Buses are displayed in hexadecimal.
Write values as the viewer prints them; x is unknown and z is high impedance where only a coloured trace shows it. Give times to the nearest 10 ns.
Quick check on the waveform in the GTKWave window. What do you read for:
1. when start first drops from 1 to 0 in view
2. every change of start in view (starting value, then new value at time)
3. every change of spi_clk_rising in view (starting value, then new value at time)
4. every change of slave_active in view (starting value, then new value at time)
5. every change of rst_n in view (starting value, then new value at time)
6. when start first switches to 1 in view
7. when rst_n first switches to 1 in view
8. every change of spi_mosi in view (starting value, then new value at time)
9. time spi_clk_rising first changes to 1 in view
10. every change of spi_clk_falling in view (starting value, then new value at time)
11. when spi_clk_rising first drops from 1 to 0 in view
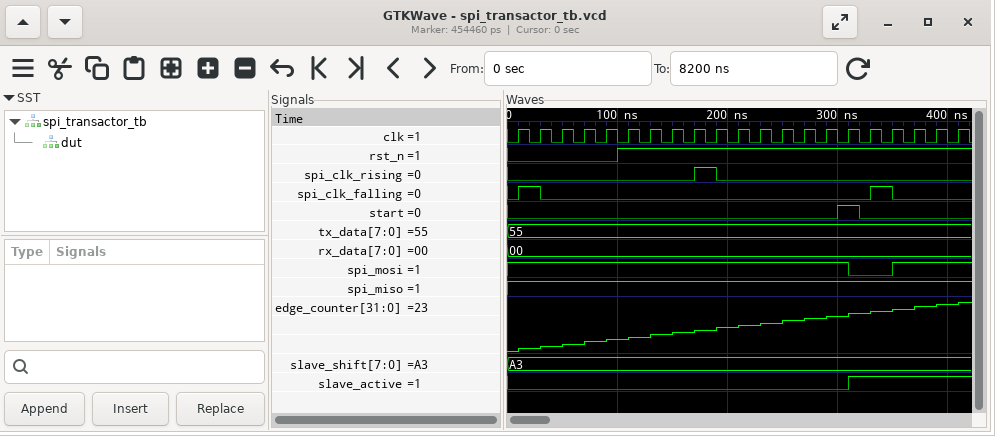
320 ns
0, 1 at 300 ns, 0 at 320 ns
0, 1 at 170 ns, 0 at 190 ns
0, 1 at 310 ns
0, 1 at 100 ns
300 ns
100 ns
1, 0 at 310 ns, 1 at 350 ns
170 ns
0, 1 at 10 ns, 0 at 30 ns, 1 at 330 ns, 0 at 350 ns
190 ns
